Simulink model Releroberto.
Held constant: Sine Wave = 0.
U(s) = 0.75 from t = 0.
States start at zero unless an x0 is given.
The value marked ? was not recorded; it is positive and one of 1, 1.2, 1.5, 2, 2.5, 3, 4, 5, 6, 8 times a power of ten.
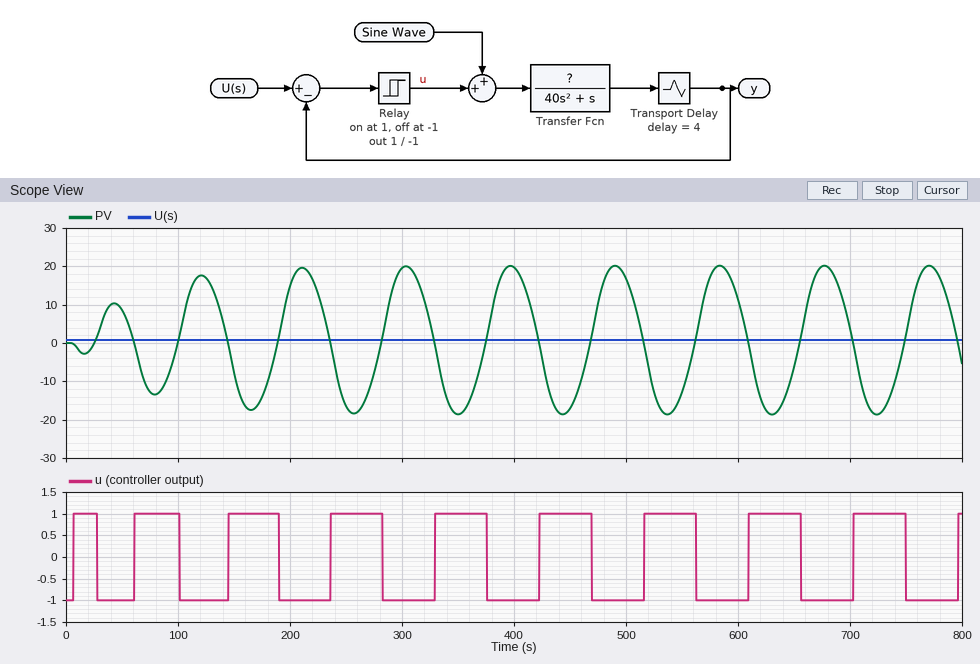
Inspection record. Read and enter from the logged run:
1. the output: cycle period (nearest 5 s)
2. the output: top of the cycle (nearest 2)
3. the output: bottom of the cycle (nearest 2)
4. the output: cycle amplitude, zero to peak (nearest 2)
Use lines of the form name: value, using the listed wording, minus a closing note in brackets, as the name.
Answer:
the output: cycle period: 95 s
the output: top of the cycle: 20
the output: bottom of the cycle: -18
the output: cycle amplitude, zero to peak: 20
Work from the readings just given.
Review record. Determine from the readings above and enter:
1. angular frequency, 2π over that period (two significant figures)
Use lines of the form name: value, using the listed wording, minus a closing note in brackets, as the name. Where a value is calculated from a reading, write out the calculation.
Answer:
angular frequency, 2π over that period: 2π / 95 = 0.066 rad/s
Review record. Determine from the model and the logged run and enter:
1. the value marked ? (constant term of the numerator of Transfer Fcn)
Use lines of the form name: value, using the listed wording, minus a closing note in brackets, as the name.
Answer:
the value marked ?: 3
